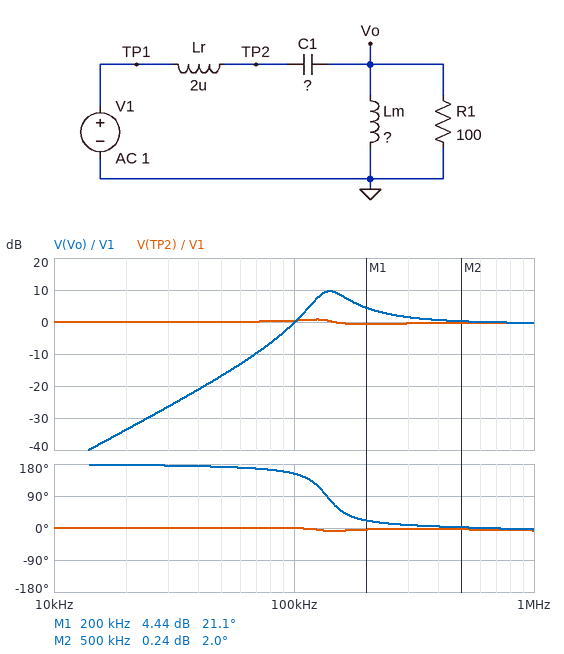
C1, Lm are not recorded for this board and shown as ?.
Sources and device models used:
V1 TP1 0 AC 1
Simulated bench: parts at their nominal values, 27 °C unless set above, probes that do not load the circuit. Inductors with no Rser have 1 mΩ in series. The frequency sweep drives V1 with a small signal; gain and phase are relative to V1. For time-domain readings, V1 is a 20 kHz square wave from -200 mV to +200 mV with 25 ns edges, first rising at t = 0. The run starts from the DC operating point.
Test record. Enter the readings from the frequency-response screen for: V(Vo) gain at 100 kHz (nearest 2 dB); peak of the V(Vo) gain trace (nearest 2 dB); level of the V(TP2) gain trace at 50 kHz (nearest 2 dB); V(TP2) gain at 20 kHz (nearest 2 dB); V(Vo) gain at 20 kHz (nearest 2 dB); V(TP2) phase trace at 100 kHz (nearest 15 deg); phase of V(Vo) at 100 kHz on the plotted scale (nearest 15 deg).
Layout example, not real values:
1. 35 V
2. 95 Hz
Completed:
1. 0 dB
2. 10 dB
3. 0 dB
4. 0 dB
5. -34 dB
6. 0 deg
7. 150 deg
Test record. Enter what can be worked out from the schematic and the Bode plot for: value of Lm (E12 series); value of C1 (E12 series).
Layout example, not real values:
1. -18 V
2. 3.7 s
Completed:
1. 39 µH
2. 33 nF
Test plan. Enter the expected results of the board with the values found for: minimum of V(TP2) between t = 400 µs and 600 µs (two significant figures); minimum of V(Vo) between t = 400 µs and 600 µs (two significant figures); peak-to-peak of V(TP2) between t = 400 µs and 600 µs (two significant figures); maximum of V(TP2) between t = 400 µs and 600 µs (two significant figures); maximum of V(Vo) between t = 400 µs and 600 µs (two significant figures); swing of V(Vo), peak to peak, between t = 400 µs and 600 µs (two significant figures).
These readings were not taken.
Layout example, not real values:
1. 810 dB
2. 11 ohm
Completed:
1. -210 mV
2. -380 mV
3. 430 mV
4. 210 mV
5. 380 mV
6. 770 mV
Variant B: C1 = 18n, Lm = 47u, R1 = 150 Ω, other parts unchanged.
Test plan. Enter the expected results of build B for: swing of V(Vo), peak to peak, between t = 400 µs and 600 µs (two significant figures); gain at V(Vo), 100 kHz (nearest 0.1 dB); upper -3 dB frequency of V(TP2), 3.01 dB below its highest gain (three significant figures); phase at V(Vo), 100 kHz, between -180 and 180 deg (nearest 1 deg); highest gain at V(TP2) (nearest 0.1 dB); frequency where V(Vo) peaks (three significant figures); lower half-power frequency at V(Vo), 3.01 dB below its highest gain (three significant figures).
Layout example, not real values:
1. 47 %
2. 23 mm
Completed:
1. 750 mV
2. -6.2 dB
3. 9.56 MHz
4. 163 deg
5. 0.7 dB
6. 174 kHz
7. 151 kHz
